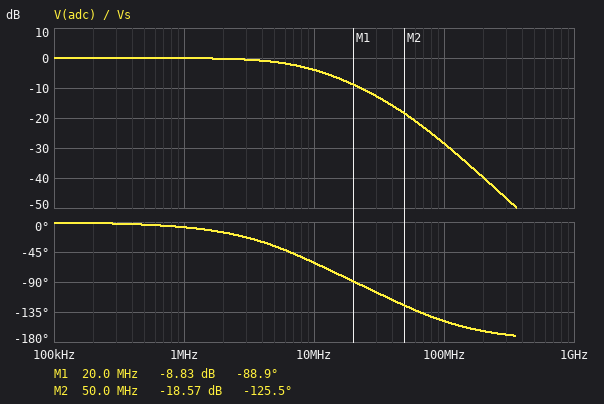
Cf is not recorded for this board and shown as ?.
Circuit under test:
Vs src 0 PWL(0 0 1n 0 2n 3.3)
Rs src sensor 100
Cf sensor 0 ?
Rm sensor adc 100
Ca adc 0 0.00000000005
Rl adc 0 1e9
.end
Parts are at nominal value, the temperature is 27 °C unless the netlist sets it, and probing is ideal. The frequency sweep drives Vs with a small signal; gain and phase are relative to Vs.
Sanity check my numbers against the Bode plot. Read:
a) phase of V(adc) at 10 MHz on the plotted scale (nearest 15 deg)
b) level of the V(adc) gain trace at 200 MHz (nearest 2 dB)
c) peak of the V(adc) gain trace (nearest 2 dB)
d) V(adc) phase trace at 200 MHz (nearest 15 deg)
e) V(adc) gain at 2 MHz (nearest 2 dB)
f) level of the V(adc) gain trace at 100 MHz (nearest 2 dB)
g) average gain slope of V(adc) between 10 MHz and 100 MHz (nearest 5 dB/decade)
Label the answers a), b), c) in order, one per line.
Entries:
a) -60 deg
b) -40 dB
c) 0 dB
d) -165 deg
e) 0 dB
f) -28 dB
g) -25 dB/decade
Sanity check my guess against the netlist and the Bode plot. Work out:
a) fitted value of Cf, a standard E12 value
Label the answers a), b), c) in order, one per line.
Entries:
a) 120 pF
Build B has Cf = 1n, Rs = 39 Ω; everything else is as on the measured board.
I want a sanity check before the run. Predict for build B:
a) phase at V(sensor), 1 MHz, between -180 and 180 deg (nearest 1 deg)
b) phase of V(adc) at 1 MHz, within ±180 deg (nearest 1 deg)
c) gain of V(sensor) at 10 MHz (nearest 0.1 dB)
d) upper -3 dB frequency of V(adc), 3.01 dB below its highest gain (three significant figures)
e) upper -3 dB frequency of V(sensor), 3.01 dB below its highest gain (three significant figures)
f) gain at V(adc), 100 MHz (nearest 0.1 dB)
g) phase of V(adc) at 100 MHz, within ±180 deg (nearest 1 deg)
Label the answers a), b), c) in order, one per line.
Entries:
a) -14 deg
b) -16 deg
c) -8.8 dB
d) 3.81 MHz
e) 3.87 MHz
f) -38.2 dB
g) -159 deg
